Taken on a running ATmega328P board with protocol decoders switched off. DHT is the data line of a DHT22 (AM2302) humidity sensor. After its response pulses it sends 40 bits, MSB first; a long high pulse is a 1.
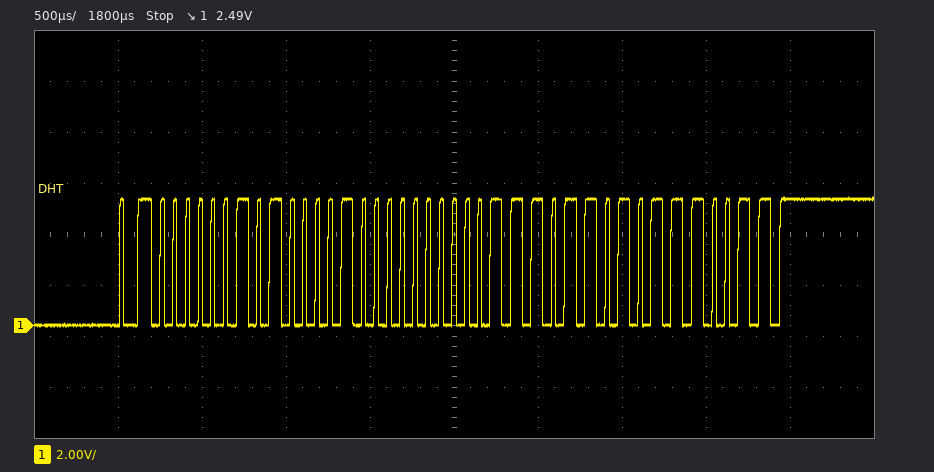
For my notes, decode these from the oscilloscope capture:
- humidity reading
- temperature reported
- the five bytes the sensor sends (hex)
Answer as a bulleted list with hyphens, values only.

- 64.4 %
- 23.7 °C
- 02 84 00 ED 73
